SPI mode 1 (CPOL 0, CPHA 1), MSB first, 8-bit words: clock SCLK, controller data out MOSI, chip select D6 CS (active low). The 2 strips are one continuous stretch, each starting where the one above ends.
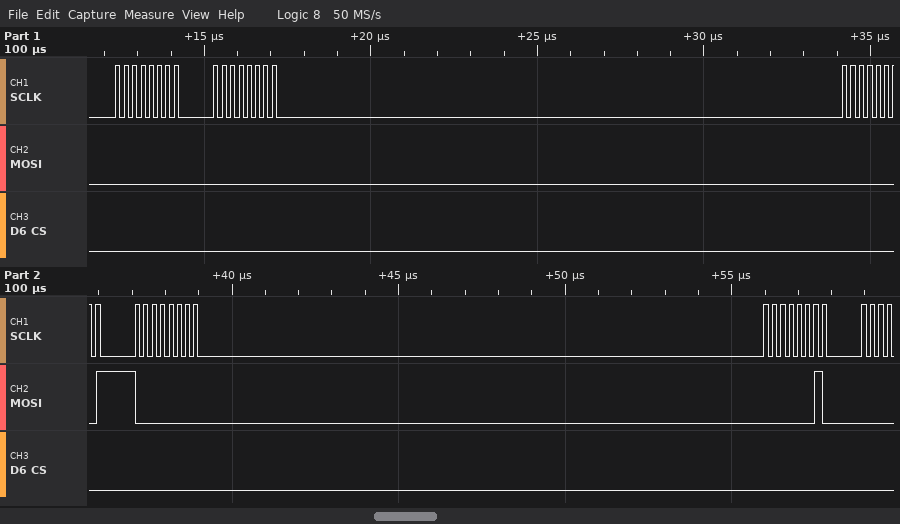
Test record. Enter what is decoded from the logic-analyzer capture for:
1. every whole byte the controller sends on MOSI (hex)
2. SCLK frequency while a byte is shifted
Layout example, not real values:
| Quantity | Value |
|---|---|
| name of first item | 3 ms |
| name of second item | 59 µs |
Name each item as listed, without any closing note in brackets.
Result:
| Quantity | Value |
|---|---|
| every whole byte the controller sends on MOSI | 00 00 01 00 02 |
| SCLK frequency while a byte is shifted | 4 MHz |
